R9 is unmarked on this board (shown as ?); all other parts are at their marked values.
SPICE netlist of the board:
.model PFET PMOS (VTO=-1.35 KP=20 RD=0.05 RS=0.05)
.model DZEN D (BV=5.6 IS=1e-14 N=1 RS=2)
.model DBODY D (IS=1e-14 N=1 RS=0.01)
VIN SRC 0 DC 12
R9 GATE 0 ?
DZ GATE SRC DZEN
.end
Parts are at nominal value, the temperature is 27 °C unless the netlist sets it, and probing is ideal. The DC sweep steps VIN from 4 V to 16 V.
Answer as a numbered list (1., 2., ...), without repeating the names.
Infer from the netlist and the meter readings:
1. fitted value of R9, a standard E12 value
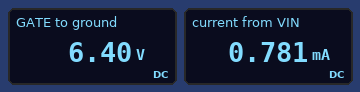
1. 8.2 kΩ
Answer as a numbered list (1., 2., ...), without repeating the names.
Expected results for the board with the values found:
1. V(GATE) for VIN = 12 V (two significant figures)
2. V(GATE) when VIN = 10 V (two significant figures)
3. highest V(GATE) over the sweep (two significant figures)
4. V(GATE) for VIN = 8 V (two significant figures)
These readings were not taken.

1. 6.4 V
2. 4.4 V
3. 10 V
4. 2.4 V
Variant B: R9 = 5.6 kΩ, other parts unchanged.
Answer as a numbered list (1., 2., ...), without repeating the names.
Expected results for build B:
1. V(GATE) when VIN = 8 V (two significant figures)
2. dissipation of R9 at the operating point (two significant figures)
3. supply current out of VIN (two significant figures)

1. 2.4 V
2. 7.3 mW
3. 1.1 mA
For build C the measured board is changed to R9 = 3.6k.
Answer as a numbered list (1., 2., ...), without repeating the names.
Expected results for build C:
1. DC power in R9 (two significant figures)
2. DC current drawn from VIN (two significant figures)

1. 11 mW
2. 1.8 mA
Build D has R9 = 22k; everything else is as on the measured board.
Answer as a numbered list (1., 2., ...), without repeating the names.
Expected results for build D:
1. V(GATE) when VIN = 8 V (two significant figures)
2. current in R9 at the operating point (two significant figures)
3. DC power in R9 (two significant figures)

1. 2.5 V
2. 290 µA
3. 1.9 mW
